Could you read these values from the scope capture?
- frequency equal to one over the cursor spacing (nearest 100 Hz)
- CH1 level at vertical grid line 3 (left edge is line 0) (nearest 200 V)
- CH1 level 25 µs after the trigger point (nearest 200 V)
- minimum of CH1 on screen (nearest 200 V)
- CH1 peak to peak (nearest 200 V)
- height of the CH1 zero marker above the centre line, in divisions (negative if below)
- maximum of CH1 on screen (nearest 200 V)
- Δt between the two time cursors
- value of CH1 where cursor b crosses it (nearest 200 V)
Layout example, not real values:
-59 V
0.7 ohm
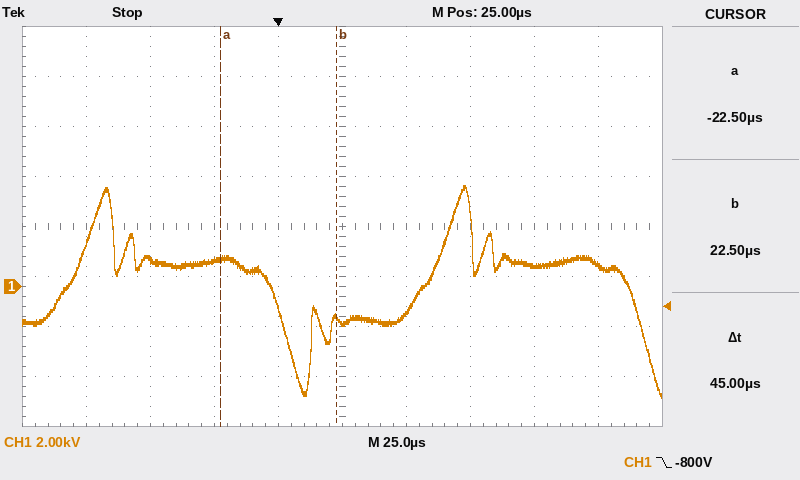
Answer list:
22.2 kHz
1.0 kV
-1.4 kV
-4.4 kV
8.4 kV
-1.2 div
4.0 kV
45 µs
-1.2 kV
